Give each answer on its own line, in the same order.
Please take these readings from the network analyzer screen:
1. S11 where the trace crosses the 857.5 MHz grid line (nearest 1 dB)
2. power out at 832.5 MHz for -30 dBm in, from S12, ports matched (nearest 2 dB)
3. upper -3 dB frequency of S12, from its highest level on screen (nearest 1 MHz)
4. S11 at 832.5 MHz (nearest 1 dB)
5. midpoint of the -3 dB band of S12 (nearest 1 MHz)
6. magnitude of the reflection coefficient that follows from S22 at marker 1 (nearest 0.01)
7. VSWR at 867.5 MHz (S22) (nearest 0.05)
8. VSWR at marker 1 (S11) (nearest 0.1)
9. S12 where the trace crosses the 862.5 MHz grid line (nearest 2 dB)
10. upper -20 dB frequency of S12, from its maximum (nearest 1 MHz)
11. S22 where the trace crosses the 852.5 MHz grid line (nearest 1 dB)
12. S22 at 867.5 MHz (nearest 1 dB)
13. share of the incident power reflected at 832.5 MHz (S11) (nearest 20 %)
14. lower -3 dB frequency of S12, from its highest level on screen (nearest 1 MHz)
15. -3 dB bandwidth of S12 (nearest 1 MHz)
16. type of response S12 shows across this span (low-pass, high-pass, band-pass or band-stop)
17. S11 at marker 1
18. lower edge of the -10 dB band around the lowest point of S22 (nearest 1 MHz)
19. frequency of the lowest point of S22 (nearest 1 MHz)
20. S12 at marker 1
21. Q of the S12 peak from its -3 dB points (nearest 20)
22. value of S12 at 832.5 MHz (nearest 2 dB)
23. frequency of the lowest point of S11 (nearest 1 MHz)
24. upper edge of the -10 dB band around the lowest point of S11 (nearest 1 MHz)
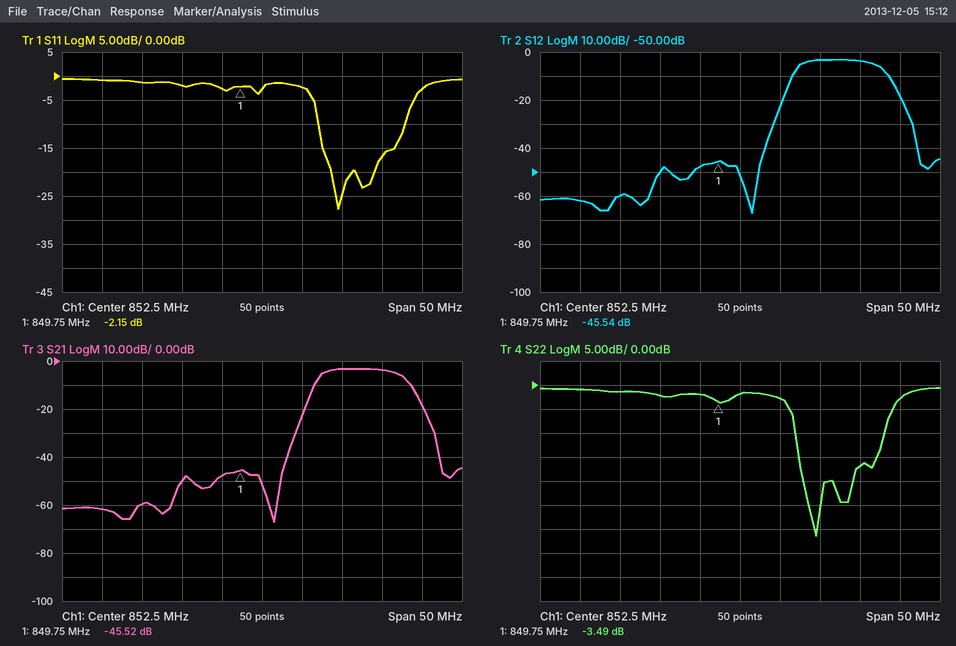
-2 dB
-92 dBm
870 MHz
-1 dB
865 MHz
0.67
1.35
8.1
-4 dB
873 MHz
-2 dB
-17 dB
80 %
860 MHz
10 MHz
band-pass
-2.15 dB
859 MHz
862 MHz
-45.54 dB
80
-62 dB
862 MHz
870 MHz
